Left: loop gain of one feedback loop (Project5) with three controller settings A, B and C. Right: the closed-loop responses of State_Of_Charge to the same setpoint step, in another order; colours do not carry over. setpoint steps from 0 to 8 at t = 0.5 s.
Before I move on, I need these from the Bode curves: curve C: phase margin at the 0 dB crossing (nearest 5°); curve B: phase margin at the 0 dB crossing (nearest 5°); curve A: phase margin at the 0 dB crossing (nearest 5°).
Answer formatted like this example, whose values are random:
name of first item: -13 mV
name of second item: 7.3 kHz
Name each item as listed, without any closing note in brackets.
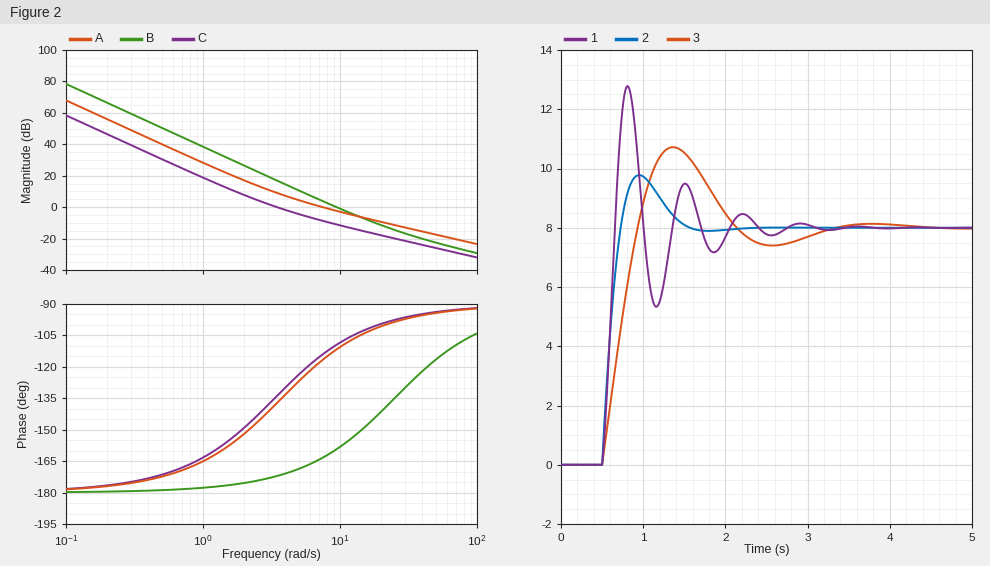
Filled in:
curve C: phase margin at the 0 dB crossing: 45°
curve B: phase margin at the 0 dB crossing: 20°
curve A: phase margin at the 0 dB crossing: 65°
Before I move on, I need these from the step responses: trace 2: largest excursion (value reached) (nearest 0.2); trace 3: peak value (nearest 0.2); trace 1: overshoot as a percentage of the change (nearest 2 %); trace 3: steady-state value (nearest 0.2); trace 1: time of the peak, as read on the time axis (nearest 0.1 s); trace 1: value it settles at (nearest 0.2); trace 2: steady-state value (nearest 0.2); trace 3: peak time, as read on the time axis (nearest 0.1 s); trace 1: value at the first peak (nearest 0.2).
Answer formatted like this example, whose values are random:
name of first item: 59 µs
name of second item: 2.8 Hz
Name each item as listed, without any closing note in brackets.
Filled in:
trace 2: largest excursion (value reached): 9.8
trace 3: peak value: 10.8
trace 1: overshoot as a percentage of the change: 60 %
trace 3: steady-state value: 8.0
trace 1: time of the peak, as read on the time axis: 0.8 s
trace 1: value it settles at: 8.0
trace 2: steady-state value: 8.0
trace 3: peak time, as read on the time axis: 1.4 s
trace 1: value at the first peak: 12.8
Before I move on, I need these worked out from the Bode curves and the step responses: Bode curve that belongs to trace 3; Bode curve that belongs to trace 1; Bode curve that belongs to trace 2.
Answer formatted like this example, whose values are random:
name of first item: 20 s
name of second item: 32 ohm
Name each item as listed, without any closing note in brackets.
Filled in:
Bode curve that belongs to trace 3: C
Bode curve that belongs to trace 1: B
Bode curve that belongs to trace 2: A
